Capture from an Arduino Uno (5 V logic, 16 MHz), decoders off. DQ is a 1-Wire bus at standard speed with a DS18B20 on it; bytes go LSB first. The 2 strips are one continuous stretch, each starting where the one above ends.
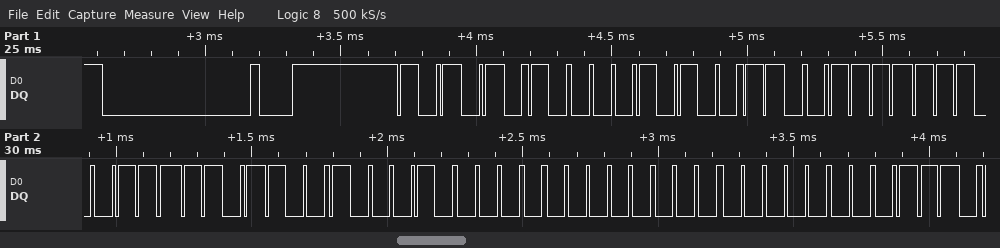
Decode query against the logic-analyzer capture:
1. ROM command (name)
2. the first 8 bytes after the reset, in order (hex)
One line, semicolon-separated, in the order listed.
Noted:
Match ROM; 55 28 F3 E7 9B 08 00 00
